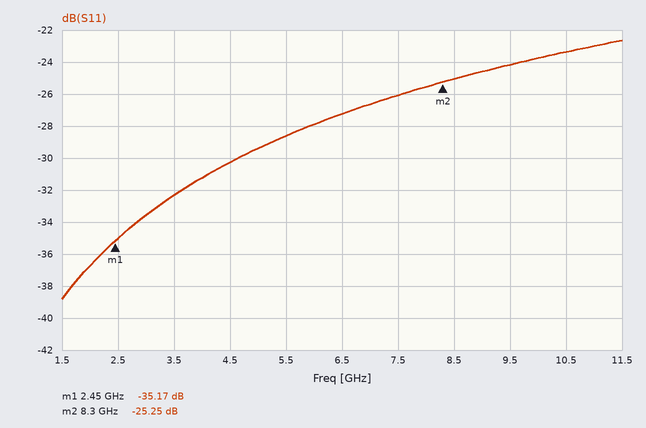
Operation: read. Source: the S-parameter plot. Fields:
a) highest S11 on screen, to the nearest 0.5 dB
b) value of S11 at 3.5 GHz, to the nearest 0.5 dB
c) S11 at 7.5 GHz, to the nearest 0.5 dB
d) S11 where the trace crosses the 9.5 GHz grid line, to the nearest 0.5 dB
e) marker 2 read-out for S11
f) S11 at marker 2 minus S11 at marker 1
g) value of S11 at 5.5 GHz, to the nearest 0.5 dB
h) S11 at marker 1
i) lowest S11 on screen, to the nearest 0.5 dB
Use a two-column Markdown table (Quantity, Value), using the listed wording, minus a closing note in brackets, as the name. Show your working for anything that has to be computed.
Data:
| Quantity | Value |
|---|---|
| highest S11 on screen, to the nearest 0.5 dB | -22.5 dB |
| value of S11 at 3.5 GHz, to the nearest 0.5 dB | -32.5 dB |
| S11 at 7.5 GHz, to the nearest 0.5 dB | -26.0 dB |
| S11 where the trace crosses the 9.5 GHz grid line, to the nearest 0.5 dB | -24.0 dB |
| marker 2 read-out for S11 | -25.25 dB |
| S11 at marker 2 minus S11 at marker 1 | -25.25 − (-35.17) = 9.92 dB |
| value of S11 at 5.5 GHz, to the nearest 0.5 dB | -28.5 dB |
| S11 at marker 1 | -35.17 dB |
| lowest S11 on screen, to the nearest 0.5 dB | -39.0 dB |
